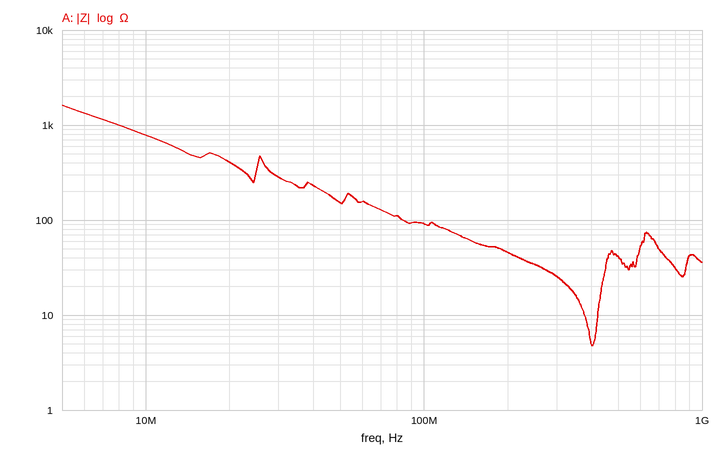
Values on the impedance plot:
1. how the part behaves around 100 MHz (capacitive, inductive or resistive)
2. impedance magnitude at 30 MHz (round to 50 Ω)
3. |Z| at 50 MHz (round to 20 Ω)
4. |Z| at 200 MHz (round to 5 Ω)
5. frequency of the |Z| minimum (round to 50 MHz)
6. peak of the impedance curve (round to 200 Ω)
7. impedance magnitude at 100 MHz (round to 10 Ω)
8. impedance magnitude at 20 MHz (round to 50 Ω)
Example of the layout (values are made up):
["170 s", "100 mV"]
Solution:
["capacitive", "300 Ω", "160 Ω", "45 Ω", "400 MHz", "1.6 kΩ", "90 Ω", "400 Ω"]
